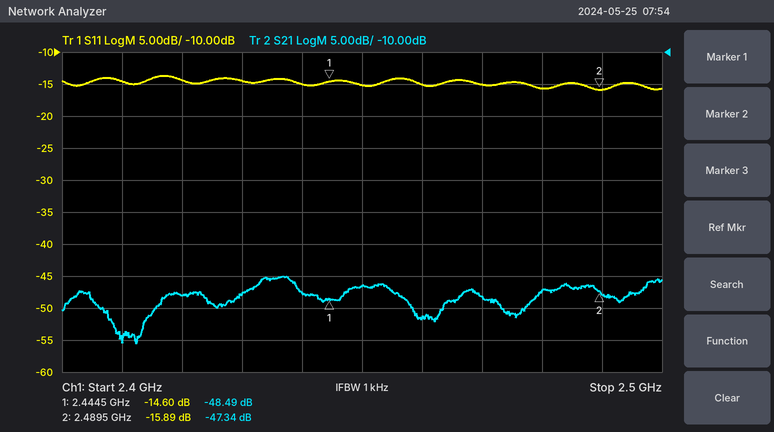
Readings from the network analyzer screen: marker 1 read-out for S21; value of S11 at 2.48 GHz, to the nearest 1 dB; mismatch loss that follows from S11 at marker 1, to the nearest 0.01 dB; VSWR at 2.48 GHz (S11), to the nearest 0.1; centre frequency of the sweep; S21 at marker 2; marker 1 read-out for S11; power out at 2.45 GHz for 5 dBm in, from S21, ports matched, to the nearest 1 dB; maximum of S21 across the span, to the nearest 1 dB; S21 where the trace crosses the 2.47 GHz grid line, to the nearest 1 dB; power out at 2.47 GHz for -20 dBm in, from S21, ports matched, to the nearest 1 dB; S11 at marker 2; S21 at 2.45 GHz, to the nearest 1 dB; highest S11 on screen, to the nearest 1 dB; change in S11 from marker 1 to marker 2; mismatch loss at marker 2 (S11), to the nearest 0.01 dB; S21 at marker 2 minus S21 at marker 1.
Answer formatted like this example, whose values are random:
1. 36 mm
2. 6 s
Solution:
1. -48.49 dB
2. -16 dB
3. 0.15 dB
4. 1.4
5. 2.45 GHz
6. -47.34 dB
7. -14.60 dB
8. -42 dBm
9. -45 dB
10. -48 dB
11. -68 dBm
12. -15.89 dB
13. -47 dB
14. -14 dB
15. -1.29 dB
16. 0.11 dB
17. 1.15 dB
